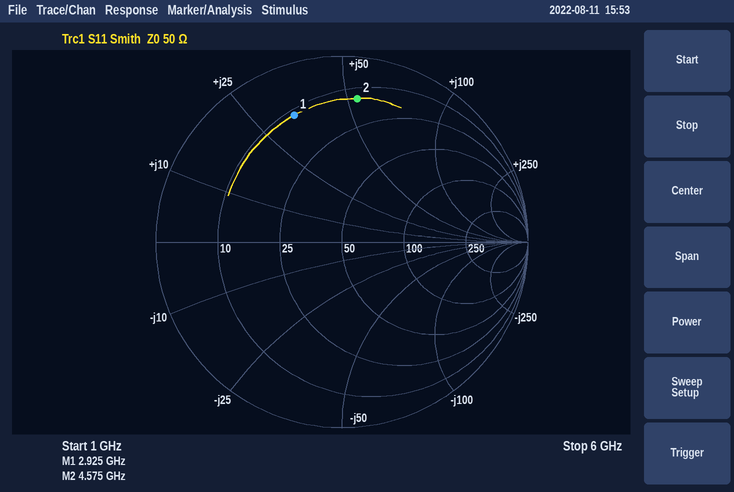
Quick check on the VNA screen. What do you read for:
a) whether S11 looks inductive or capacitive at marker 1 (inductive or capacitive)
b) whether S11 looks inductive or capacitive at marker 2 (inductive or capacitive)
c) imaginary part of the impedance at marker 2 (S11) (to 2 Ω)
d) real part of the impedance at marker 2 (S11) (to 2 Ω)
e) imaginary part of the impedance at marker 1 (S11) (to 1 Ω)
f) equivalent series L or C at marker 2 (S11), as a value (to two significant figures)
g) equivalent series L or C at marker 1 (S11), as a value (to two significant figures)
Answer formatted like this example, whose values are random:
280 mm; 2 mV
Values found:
inductive; inductive; +54 Ω; 14 Ω; +33 Ω; 1.9 nH; 1.8 nH
